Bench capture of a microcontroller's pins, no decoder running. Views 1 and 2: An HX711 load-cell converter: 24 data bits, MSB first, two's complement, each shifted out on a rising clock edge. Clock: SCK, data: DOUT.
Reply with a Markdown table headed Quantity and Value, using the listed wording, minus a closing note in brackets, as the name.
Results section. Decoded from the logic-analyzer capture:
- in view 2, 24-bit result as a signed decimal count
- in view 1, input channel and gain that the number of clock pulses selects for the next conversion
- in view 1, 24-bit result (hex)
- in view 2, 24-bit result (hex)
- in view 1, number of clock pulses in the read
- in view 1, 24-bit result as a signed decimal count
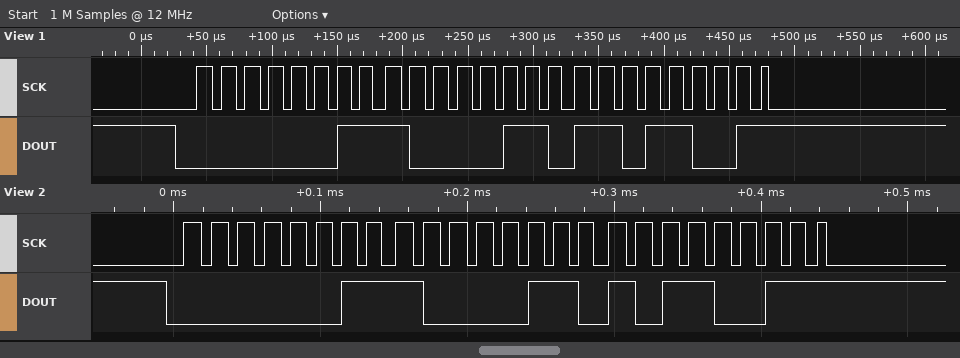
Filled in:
| Quantity | Value |
|---|---|
| in view 2, 24-bit result as a signed decimal count | 231091 |
| in view 1, input channel and gain that the number of clock pulses selects for the next conversion | channel A, gain 128 |
| in view 1, 24-bit result | 0x0386D9 |
| in view 2, 24-bit result | 0x0386B3 |
| in view 1, number of clock pulses in the read | 25 |
| in view 1, 24-bit result as a signed decimal count | 231129 |
